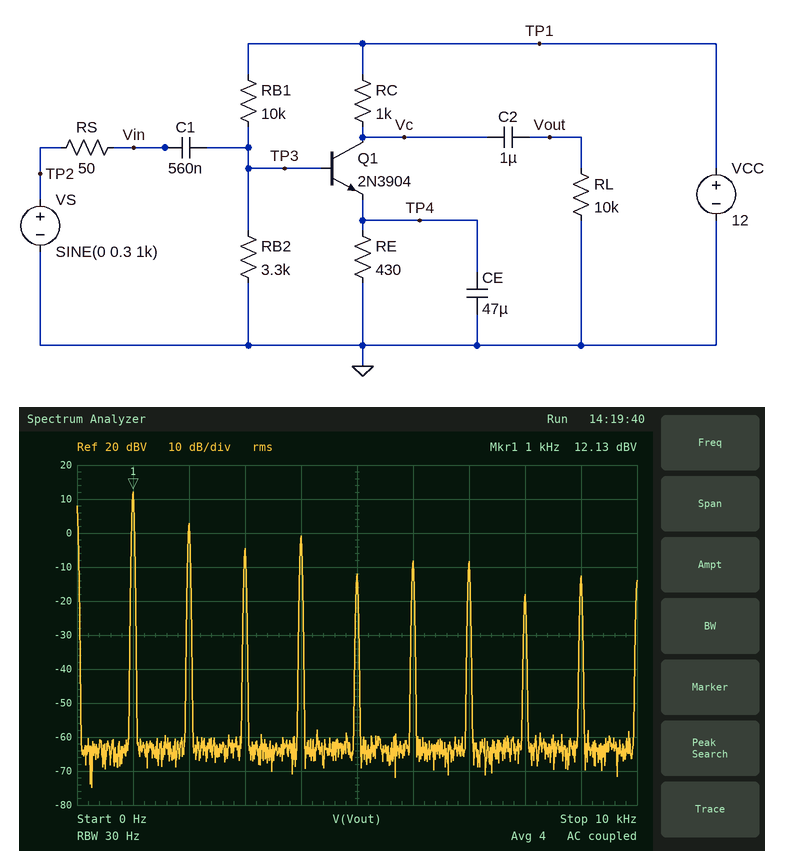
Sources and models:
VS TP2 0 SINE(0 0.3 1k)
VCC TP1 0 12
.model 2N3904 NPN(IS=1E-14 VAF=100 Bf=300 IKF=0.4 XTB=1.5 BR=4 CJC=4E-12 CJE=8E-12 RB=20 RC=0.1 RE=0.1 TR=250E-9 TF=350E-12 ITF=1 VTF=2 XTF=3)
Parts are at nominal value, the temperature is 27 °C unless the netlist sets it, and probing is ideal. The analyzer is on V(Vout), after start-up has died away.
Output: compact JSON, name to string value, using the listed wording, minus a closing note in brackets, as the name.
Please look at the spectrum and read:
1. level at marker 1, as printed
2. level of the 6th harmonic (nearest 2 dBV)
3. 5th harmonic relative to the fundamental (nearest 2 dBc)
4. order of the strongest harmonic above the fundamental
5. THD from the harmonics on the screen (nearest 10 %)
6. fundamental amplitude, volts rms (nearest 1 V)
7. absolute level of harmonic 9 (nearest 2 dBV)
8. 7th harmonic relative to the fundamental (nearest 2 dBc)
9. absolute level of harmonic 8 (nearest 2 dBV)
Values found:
{"level at marker 1, as printed": "12.13 dBV", "level of the 6th harmonic": "-8 dBV", "5th harmonic relative to the fundamental": "-24 dBc", "order of the strongest harmonic above the fundamental": "2", "THD from the harmonics on the screen": "50 %", "fundamental amplitude, volts rms": "4 V", "absolute level of harmonic 9": "-12 dBV", "7th harmonic relative to the fundamental": "-20 dBc", "absolute level of harmonic 8": "-18 dBV"}
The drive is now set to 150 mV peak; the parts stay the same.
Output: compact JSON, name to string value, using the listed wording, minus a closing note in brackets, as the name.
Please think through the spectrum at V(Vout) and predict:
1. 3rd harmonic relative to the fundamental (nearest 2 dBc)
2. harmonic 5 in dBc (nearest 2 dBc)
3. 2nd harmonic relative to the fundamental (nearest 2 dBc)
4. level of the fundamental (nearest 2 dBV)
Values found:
{"3rd harmonic relative to the fundamental": "-14 dBc", "harmonic 5 in dBc": "-26 dBc", "2nd harmonic relative to the fundamental": "-14 dBc", "level of the fundamental": "12 dBV"}
